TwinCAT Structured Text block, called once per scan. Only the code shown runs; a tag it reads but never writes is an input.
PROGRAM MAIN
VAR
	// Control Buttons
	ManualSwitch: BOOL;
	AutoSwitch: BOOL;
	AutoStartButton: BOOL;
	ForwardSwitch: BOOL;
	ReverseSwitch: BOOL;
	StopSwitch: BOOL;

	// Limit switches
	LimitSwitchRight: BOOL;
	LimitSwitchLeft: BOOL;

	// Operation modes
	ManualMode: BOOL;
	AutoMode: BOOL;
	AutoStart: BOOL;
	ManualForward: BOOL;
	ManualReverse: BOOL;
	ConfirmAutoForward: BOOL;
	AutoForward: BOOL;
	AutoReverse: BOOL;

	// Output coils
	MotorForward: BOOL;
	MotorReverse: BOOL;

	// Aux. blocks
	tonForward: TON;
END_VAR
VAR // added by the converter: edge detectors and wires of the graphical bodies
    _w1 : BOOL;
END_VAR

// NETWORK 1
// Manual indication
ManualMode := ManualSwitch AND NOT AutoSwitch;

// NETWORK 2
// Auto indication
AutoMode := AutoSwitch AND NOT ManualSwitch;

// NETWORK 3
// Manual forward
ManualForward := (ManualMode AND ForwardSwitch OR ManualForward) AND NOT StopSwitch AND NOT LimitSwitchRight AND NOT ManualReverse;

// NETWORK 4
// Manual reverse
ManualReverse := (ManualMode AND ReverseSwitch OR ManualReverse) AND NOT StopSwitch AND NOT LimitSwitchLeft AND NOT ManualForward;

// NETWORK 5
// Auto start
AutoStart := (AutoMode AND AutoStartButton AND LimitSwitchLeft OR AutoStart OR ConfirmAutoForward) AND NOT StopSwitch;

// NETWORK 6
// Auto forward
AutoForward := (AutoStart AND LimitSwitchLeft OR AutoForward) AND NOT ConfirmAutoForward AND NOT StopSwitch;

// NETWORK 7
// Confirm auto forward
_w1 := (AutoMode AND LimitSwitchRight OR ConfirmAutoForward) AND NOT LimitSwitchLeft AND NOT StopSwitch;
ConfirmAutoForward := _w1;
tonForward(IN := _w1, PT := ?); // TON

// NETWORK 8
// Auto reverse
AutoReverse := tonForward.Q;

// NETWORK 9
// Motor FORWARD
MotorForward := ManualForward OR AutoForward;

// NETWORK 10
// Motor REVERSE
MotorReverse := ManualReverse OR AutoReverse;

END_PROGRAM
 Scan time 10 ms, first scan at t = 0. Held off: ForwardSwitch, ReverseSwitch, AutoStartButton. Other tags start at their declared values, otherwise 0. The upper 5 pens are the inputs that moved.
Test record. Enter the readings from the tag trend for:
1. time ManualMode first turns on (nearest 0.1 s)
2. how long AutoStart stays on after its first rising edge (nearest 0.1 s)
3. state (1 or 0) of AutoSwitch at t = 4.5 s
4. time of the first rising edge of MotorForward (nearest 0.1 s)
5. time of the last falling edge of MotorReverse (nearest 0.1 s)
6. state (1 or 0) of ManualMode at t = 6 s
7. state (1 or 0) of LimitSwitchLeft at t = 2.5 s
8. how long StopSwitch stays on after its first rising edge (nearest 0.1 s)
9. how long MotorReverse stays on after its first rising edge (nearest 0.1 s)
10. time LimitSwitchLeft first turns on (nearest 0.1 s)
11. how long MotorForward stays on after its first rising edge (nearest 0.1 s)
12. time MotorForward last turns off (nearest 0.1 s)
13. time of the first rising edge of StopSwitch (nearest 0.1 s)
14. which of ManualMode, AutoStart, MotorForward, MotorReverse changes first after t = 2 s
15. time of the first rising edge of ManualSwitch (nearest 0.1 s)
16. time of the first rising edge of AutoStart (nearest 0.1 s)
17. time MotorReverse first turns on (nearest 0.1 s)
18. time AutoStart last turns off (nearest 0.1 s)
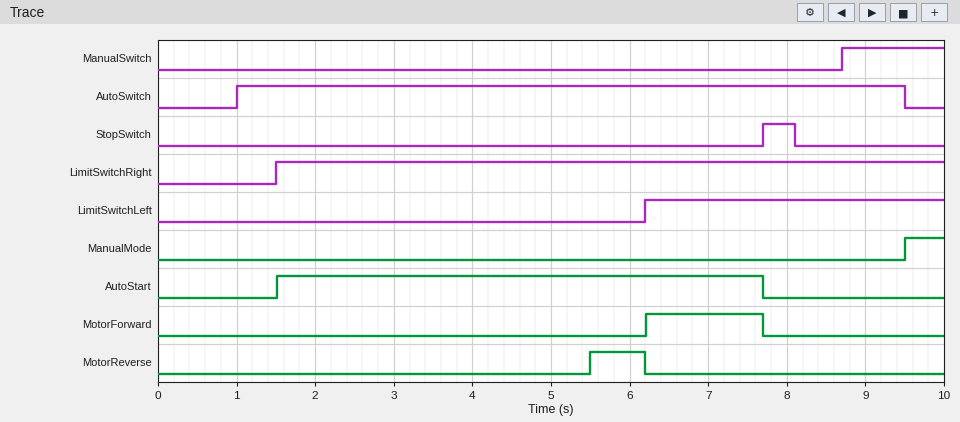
9.5 s
6.2 s
1
6.2 s
6.2 s
0
0
0.4 s
0.7 s
6.2 s
1.5 s
7.7 s
7.7 s
MotorReverse
8.7 s
1.5 s
5.5 s
7.7 s
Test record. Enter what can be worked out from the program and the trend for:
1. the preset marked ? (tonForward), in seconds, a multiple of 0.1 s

4.0 s
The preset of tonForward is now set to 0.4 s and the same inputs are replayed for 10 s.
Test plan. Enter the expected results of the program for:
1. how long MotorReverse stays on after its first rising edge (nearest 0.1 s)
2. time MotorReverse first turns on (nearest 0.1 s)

4.3 s
1.9 s
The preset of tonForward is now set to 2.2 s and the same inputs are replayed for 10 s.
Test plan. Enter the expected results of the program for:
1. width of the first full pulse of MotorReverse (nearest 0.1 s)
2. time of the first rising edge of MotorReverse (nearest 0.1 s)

2.5 s
3.7 s
